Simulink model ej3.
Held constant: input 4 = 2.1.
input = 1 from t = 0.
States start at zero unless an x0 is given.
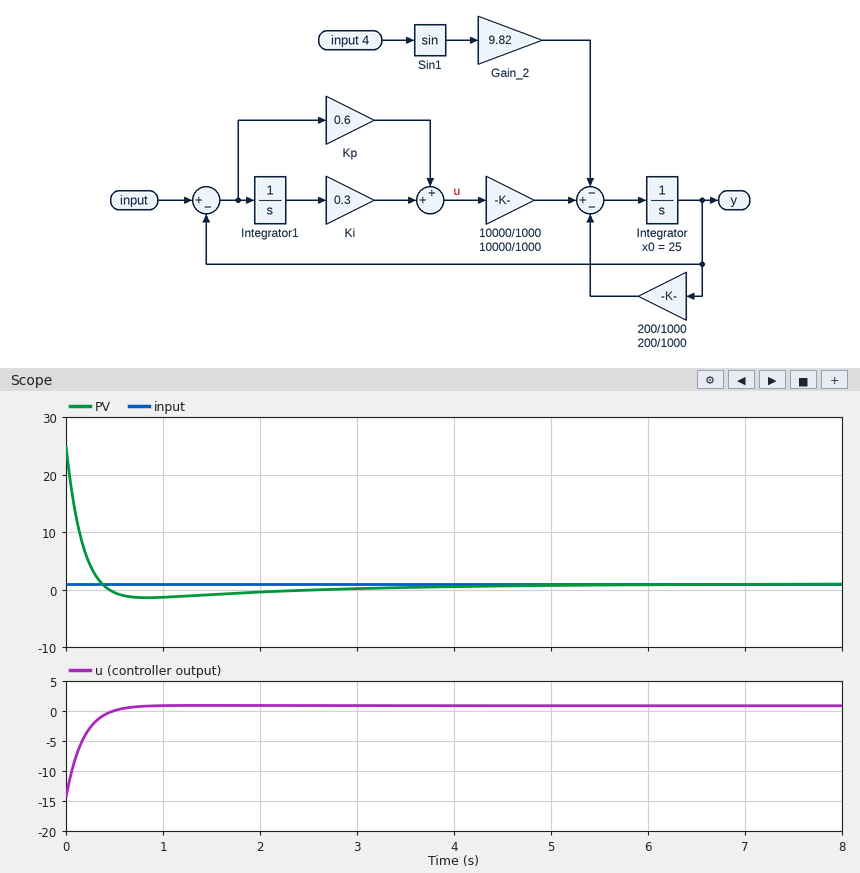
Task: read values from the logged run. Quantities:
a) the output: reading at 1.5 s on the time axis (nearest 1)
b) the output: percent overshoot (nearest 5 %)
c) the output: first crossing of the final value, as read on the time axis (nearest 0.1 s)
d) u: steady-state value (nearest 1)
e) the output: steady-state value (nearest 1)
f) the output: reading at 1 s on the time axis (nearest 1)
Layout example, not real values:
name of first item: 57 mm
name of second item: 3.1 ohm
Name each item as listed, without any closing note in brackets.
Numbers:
the output: reading at 1.5 s on the time axis: -1
the output: percent overshoot: 10 %
the output: first crossing of the final value, as read on the time axis: 0.4 s
u: steady-state value: 1
the output: steady-state value: 1
the output: reading at 1 s on the time axis: -1
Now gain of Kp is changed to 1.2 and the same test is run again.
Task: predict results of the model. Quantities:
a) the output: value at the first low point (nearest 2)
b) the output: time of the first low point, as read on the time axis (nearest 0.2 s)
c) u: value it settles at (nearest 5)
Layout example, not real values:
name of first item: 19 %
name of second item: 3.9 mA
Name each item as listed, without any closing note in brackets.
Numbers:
the output: value at the first low point: 0
the output: time of the first low point, as read on the time axis: 0.6 s
u: value it settles at: 0
